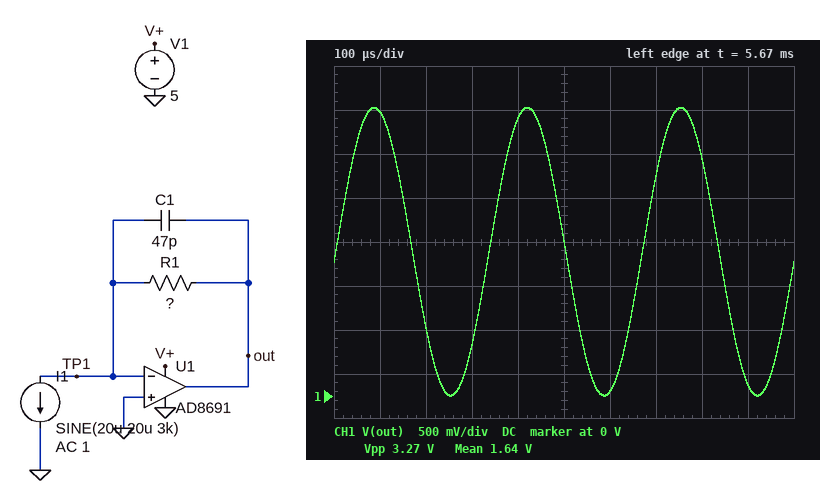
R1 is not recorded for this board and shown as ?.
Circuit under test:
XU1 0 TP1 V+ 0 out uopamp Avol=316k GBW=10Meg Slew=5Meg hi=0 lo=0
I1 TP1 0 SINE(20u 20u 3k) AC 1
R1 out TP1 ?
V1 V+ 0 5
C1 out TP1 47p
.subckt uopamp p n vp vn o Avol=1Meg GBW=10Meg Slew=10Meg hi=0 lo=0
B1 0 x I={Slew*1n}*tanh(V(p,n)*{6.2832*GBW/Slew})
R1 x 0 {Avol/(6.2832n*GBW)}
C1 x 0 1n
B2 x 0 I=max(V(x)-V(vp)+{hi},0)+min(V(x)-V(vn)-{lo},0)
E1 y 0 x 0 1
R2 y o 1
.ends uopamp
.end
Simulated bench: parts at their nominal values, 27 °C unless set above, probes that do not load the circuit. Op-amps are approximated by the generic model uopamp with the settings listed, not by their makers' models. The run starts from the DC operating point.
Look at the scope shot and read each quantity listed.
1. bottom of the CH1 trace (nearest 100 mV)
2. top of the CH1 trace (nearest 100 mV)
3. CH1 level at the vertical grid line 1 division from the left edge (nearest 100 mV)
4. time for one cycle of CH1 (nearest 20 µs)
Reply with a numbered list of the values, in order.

1. 0 V
2. 3.3 V
3. 3.2 V
4. 340 µs
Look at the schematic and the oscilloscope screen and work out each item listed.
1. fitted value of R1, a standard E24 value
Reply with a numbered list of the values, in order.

1. 82 kΩ
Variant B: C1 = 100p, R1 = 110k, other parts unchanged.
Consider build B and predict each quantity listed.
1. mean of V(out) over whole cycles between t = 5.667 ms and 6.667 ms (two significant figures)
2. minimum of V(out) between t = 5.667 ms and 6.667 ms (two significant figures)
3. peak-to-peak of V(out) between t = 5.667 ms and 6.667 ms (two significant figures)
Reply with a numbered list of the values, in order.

1. 2.2 V
2. 46 mV
3. 4.3 V
